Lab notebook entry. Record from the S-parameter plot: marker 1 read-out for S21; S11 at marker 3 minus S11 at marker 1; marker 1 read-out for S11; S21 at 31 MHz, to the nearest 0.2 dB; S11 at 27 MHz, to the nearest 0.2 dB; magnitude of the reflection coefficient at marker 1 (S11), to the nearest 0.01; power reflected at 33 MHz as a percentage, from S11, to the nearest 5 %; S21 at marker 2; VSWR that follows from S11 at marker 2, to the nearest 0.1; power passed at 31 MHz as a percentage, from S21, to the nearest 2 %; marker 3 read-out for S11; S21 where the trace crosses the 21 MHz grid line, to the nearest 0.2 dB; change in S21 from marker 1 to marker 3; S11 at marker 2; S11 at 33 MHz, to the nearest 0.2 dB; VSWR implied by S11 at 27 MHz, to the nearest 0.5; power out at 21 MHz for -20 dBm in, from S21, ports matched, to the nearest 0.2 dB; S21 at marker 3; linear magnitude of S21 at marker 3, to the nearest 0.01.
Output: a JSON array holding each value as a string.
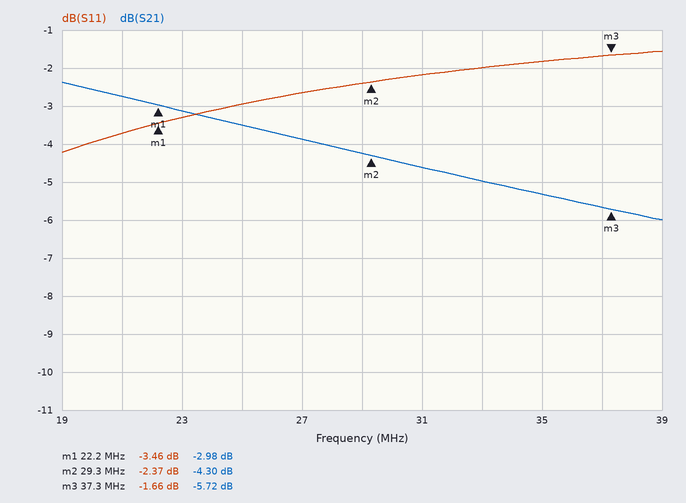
["-2.98 dB", "1.80 dB", "-3.46 dB", "-4.6 dB", "-2.6 dB", "0.67", "65 %", "-4.30 dB", "7.4", "34 %", "-1.66 dB", "-2.8 dB", "-2.74 dB", "-2.37 dB", "-2.0 dB", "6.5", "-22.8 dBm", "-5.72 dB", "0.52"]
